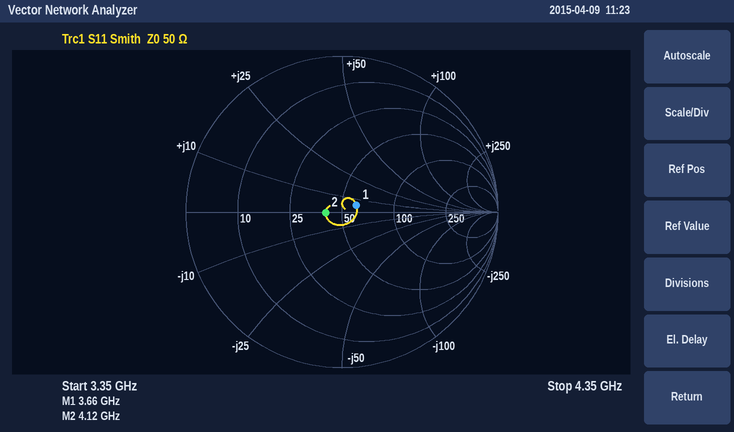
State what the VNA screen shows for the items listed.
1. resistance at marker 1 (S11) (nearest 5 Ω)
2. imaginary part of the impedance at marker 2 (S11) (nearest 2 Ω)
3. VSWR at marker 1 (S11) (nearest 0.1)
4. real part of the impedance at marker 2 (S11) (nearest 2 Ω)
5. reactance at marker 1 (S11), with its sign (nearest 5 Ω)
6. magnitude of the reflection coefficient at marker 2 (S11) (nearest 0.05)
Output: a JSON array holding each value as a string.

["60 Ω", "0 Ω", "1.2", "40 Ω", "+5 Ω", "0.10"]
